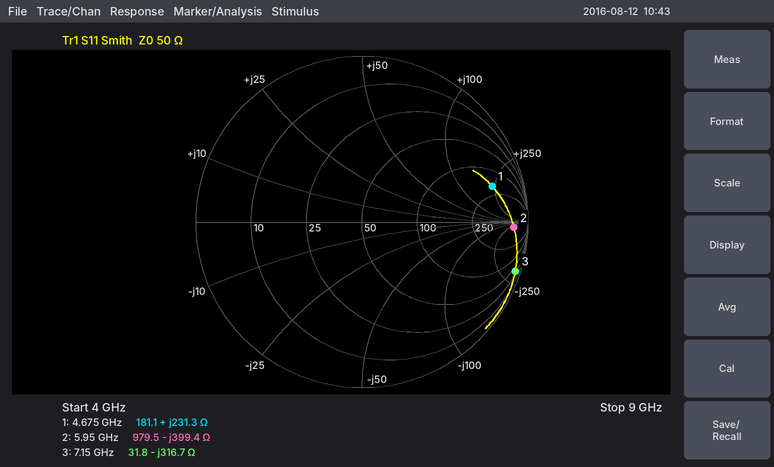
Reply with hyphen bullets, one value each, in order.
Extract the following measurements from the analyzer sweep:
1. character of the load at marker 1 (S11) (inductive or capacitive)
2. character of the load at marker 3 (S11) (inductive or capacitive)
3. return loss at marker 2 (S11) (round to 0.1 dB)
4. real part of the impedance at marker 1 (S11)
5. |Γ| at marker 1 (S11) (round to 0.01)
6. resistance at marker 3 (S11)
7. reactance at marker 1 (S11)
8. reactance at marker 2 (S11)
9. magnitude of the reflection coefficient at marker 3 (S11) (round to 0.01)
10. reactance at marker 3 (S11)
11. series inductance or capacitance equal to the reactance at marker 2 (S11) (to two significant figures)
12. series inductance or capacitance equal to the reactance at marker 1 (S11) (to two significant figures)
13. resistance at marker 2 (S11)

- inductive
- capacitive
- 0.8 dB
- 181.1 Ω
- 0.81
- 31.8 Ω
- +231.3 Ω
- -399.4 Ω
- 0.97
- -316.7 Ω
- 67 fF
- 7.9 nH
- 979.5 Ω
